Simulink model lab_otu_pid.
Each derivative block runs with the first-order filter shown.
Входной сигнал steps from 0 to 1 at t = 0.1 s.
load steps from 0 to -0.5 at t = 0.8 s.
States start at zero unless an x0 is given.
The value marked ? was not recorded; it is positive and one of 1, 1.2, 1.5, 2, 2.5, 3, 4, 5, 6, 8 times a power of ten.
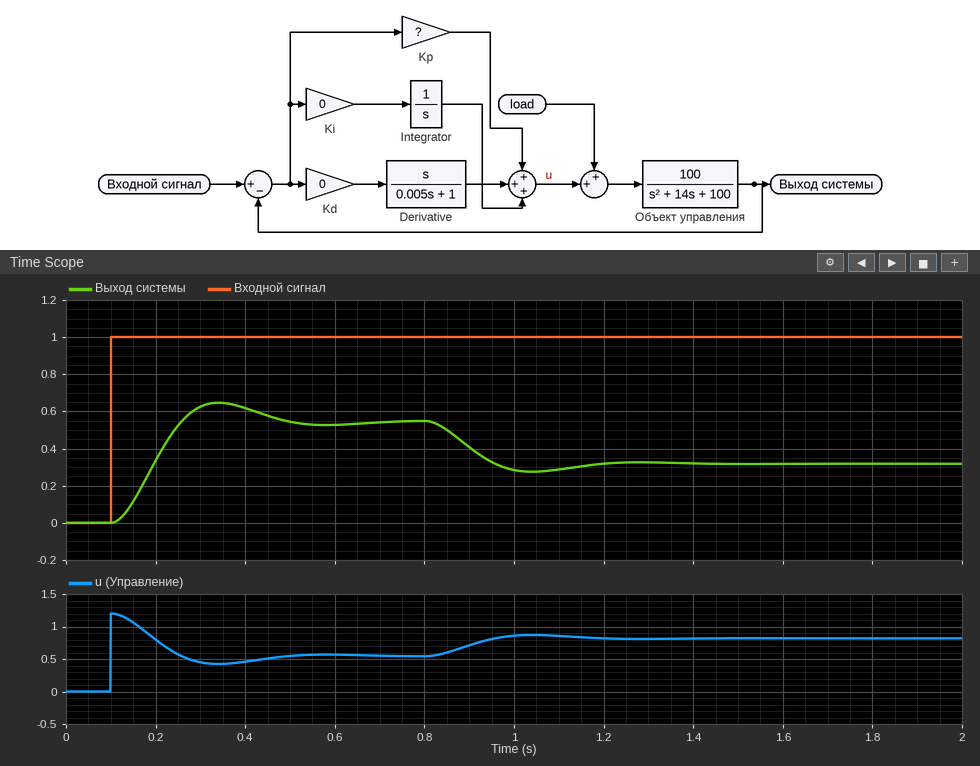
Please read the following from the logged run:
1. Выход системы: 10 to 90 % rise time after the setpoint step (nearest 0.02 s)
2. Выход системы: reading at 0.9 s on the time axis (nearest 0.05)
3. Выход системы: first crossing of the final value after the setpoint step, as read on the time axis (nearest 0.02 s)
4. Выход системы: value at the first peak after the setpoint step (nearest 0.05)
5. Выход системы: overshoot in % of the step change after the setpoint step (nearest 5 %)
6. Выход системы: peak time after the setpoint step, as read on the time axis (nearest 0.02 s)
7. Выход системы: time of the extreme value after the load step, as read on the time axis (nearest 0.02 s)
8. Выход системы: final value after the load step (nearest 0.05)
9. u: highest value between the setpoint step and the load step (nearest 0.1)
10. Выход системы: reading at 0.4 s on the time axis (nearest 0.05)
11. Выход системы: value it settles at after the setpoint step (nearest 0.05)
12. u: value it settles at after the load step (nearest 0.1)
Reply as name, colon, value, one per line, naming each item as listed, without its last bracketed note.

Выход системы: 10 to 90 % rise time after the setpoint step: 0.10 s
Выход системы: reading at 0.9 s on the time axis: 0.40
Выход системы: first crossing of the final value after the setpoint step, as read on the time axis: 0.26 s
Выход системы: value at the first peak after the setpoint step: 0.65
Выход системы: overshoot in % of the step change after the setpoint step: 20 %
Выход системы: peak time after the setpoint step, as read on the time axis: 0.34 s
Выход системы: time of the extreme value after the load step, as read on the time axis: 1.04 s
Выход системы: final value after the load step: 0.30
u: highest value between the setpoint step and the load step: 1.2
Выход системы: reading at 0.4 s on the time axis: 0.60
Выход системы: value it settles at after the setpoint step: 0.55
u: value it settles at after the load step: 0.8
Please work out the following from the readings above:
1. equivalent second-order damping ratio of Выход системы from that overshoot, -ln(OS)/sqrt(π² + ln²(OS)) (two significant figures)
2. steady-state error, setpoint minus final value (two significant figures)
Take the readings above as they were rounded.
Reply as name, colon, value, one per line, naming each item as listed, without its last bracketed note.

equivalent second-order damping ratio of Выход системы from that overshoot, -ln(OS)/sqrt(π² + ln²(OS)): 0.46
steady-state error, setpoint minus final value: 0.45
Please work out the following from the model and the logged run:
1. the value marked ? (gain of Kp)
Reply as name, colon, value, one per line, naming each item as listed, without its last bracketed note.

the value marked ?: 1.2
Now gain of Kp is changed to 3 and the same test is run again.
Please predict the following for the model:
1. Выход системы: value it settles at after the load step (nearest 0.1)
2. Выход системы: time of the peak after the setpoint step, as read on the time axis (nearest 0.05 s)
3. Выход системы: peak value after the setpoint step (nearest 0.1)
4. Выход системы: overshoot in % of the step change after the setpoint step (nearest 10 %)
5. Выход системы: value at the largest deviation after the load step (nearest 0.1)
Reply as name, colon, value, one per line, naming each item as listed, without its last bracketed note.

Выход системы: value it settles at after the load step: 0.6
Выход системы: time of the peak after the setpoint step, as read on the time axis: 0.25 s
Выход системы: peak value after the setpoint step: 1.0
Выход системы: overshoot in % of the step change after the setpoint step: 30 %
Выход системы: value at the largest deviation after the load step: 0.6
